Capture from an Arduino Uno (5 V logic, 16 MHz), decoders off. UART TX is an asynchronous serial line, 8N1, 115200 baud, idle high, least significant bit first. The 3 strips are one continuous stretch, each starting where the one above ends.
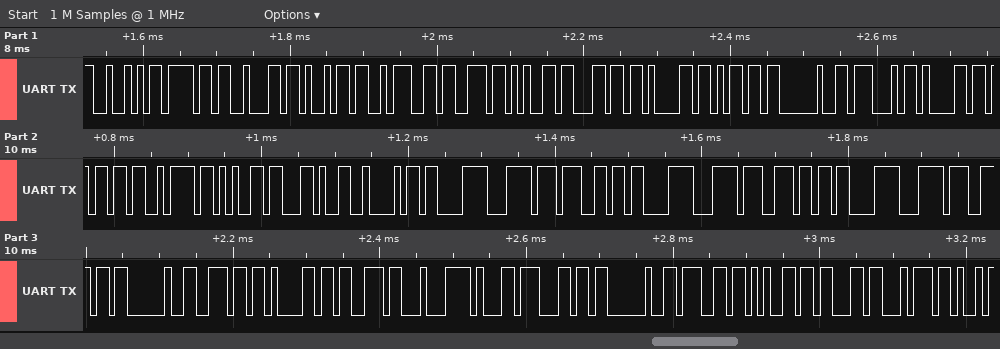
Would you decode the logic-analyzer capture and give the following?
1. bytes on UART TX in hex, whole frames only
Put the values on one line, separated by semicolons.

52 6F 62 69 3A 73 65 6C 61 6D 20 47 61 6D 7A 65 2C 42 C3 BC 67 C3 BC 6E C3 BC 6E 20 6E 61 73 C4 B1 6C 20 67 65 63 74
